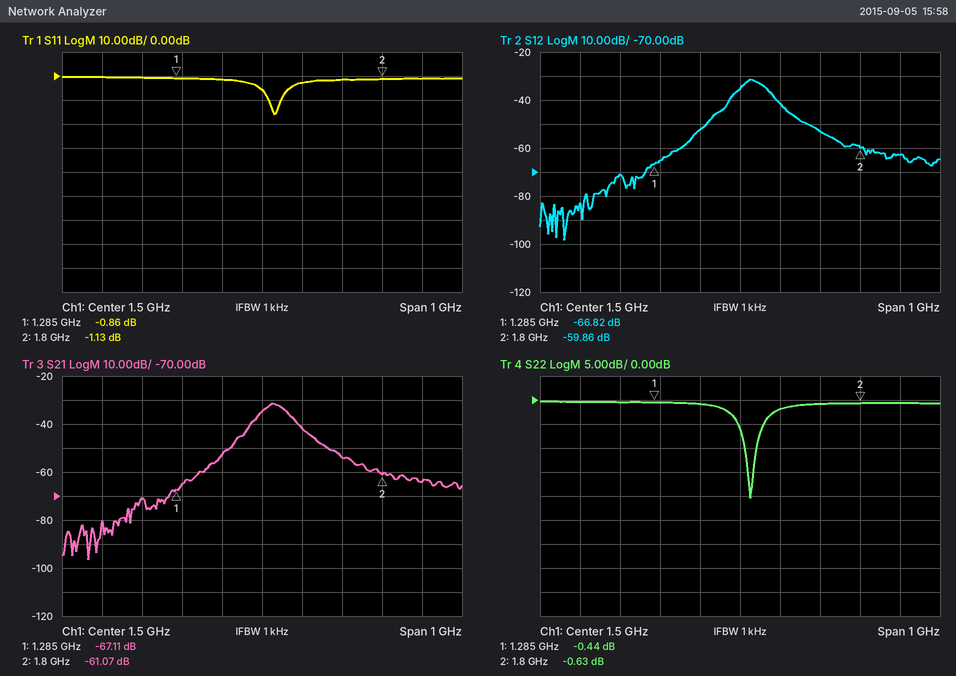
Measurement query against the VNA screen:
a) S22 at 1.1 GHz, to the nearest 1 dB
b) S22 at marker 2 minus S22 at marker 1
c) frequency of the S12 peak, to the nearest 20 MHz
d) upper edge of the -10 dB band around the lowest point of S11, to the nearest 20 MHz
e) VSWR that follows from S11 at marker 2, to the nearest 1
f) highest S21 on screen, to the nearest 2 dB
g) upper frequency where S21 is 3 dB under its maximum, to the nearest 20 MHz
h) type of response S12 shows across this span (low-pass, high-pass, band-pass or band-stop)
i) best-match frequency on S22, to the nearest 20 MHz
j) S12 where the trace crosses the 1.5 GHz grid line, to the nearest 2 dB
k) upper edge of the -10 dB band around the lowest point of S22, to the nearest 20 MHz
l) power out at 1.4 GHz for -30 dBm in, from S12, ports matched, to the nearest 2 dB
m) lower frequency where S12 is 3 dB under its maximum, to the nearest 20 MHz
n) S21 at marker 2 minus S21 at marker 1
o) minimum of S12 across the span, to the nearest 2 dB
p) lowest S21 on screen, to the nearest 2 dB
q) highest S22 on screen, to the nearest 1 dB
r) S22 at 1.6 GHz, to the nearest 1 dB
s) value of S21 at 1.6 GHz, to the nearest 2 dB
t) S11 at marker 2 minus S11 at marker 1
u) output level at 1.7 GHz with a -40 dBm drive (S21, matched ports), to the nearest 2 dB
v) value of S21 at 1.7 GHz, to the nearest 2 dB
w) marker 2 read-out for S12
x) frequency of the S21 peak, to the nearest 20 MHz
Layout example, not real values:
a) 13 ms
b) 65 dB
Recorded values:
a) 0 dB
b) -0.19 dB
c) 1.52 GHz
d) 1.54 GHz
e) 15
f) -32 dB
g) 1.56 GHz
h) band-pass
i) 1.52 GHz
j) -36 dB
k) 1.54 GHz
l) -82 dBm
m) 1.50 GHz
n) 6.04 dB
o) -98 dB
p) -96 dB
q) 0 dB
r) -2 dB
s) -42 dB
t) -0.27 dB
u) -94 dBm
v) -54 dB
w) -59.86 dB
x) 1.52 GHz
